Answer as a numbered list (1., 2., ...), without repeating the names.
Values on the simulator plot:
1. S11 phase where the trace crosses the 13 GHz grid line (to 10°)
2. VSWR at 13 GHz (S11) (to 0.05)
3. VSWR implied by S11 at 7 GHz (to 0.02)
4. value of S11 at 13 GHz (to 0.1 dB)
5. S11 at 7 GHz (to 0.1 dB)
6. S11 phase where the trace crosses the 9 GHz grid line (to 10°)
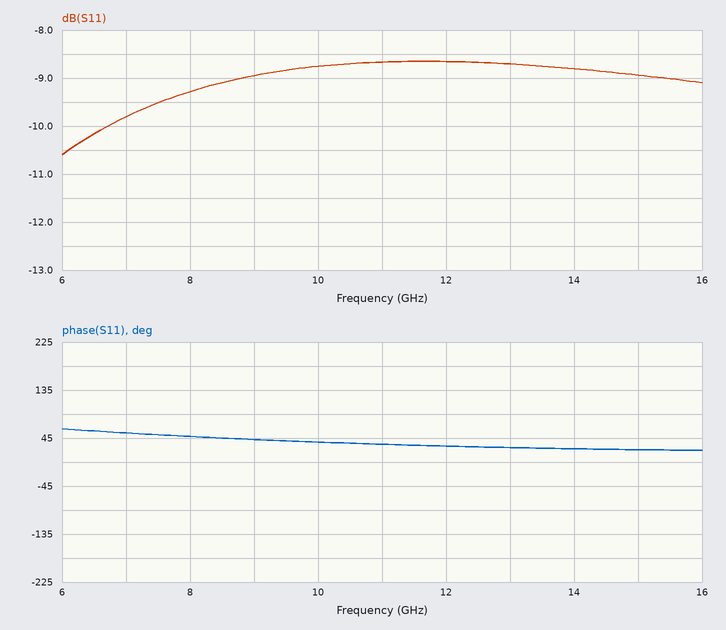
1. 30°
2. 2.15
3. 1.96
4. -8.7 dB
5. -9.8 dB
6. 40°
